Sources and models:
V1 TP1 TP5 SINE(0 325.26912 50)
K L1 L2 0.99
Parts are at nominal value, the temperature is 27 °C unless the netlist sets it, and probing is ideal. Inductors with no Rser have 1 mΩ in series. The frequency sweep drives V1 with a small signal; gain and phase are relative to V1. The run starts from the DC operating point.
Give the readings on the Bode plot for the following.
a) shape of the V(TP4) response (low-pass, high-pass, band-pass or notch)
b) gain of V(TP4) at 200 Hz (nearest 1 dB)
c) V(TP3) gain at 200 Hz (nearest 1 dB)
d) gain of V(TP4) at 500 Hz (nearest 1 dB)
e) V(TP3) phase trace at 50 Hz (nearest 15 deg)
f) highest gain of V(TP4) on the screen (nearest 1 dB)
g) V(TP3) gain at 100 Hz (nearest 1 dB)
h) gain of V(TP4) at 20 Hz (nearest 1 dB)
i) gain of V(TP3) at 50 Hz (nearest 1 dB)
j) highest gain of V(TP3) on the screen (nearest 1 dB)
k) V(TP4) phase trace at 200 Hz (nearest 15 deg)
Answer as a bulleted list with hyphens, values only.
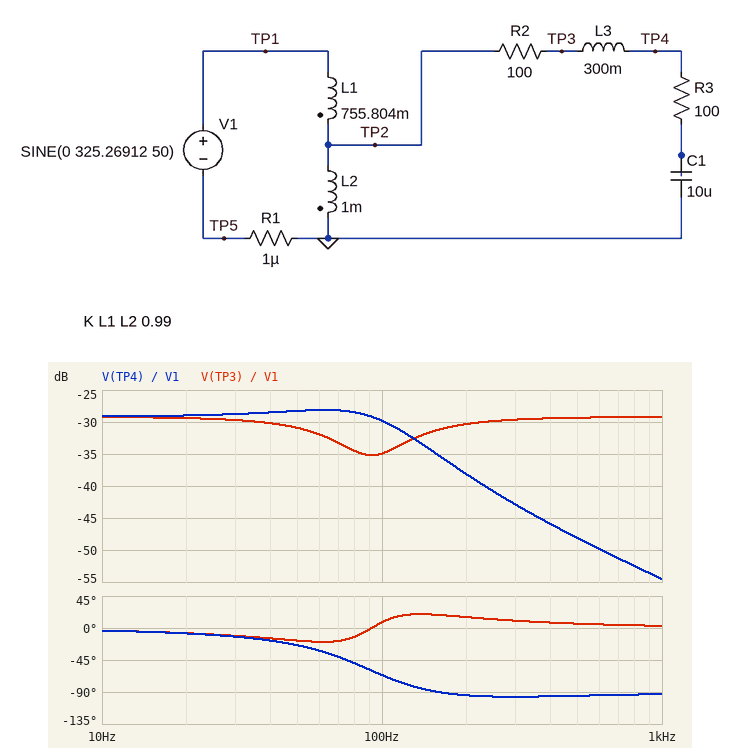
- low-pass
- -38 dB
- -30 dB
- -48 dB
- -15 deg
- -28 dB
- -35 dB
- -29 dB
- -31 dB
- -29 dB
- -90 deg
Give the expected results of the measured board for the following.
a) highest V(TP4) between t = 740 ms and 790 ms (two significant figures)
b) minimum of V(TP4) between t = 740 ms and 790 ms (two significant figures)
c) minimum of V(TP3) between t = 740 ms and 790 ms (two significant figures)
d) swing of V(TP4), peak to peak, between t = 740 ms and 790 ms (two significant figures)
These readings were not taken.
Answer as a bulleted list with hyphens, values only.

- 13 V
- -13 V
- -9.2 V
- 25 V
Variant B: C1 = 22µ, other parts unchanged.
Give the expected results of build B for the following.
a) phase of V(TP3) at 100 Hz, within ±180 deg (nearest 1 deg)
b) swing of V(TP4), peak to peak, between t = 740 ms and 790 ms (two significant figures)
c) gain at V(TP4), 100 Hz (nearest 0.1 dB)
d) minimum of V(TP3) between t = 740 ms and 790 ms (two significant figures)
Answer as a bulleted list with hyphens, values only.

- 19 deg
- 19 V
- -34.6 dB
- -6.1 V
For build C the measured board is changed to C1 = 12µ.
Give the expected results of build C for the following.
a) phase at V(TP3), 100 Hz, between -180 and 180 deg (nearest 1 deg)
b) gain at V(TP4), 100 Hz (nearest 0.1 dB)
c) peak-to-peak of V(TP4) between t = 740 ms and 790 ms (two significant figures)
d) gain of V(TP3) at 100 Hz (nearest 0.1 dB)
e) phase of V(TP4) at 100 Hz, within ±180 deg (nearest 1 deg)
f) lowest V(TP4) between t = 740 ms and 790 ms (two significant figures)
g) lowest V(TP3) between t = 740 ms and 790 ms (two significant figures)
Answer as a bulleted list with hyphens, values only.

- 14 deg
- -31.1 dB
- 24 V
- -34.3 dB
- -69 deg
- -12 V
- -8.5 V
